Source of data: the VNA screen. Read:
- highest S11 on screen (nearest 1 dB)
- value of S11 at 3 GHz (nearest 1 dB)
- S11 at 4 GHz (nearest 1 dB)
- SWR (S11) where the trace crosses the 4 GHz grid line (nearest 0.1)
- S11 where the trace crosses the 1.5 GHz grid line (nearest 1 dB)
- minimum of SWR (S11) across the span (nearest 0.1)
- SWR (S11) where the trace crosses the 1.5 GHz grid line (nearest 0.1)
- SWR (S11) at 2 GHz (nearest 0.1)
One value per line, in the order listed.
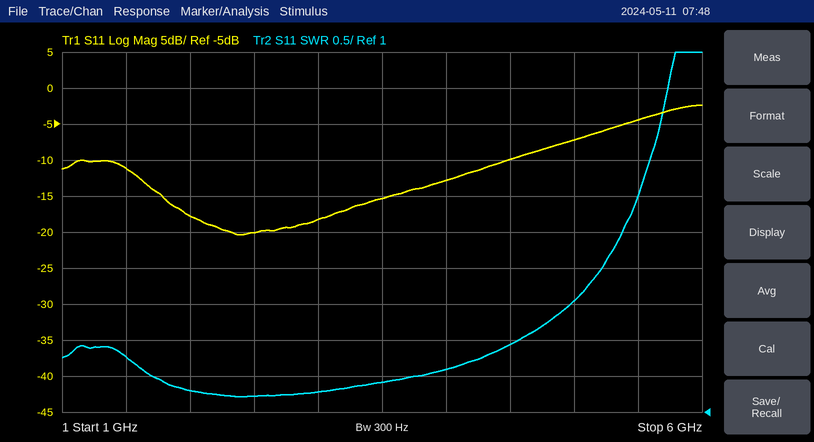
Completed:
-2 dB
-18 dB
-13 dB
1.6
-11 dB
1.2
1.8
1.3
